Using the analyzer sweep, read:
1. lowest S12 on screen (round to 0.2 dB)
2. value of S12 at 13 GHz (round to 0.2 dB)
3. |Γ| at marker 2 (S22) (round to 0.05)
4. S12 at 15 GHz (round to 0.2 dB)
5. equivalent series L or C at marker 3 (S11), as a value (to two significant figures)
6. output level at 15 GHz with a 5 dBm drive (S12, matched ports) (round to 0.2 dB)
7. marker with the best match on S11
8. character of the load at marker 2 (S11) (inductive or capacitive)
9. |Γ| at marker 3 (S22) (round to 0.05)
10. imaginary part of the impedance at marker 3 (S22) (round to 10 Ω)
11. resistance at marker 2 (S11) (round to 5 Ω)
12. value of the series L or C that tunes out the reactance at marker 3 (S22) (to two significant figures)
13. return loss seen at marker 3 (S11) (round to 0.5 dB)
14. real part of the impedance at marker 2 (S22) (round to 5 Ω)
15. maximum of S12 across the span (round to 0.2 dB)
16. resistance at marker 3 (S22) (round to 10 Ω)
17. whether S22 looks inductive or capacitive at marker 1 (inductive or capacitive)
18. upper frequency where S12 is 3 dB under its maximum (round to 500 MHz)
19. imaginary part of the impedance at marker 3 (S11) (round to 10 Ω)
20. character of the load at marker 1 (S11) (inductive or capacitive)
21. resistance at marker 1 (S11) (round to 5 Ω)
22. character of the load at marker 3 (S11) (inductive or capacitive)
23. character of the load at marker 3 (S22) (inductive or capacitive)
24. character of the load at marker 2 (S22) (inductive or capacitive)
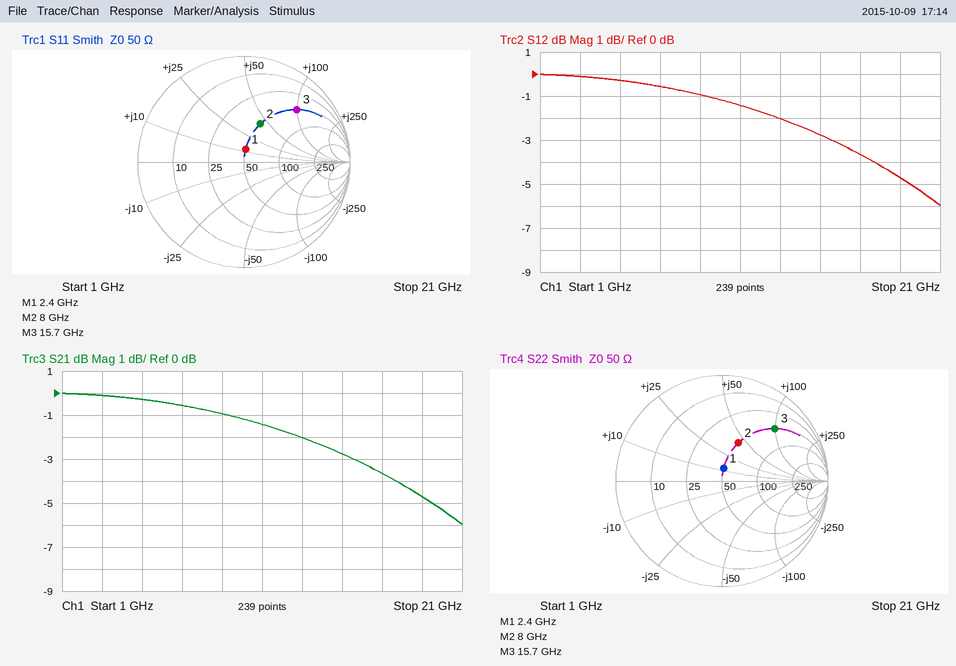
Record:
-6.0 dB
-2.0 dB
0.40
-2.8 dB
1.0 nH
2.2 dBm
marker 1
inductive
0.70
+100 Ω
50 Ω
100 fF
3.0 dB
50 Ω
0.0 dB
50 Ω
inductive
15.5 GHz
+100 Ω
inductive
50 Ω
inductive
inductive
inductive
